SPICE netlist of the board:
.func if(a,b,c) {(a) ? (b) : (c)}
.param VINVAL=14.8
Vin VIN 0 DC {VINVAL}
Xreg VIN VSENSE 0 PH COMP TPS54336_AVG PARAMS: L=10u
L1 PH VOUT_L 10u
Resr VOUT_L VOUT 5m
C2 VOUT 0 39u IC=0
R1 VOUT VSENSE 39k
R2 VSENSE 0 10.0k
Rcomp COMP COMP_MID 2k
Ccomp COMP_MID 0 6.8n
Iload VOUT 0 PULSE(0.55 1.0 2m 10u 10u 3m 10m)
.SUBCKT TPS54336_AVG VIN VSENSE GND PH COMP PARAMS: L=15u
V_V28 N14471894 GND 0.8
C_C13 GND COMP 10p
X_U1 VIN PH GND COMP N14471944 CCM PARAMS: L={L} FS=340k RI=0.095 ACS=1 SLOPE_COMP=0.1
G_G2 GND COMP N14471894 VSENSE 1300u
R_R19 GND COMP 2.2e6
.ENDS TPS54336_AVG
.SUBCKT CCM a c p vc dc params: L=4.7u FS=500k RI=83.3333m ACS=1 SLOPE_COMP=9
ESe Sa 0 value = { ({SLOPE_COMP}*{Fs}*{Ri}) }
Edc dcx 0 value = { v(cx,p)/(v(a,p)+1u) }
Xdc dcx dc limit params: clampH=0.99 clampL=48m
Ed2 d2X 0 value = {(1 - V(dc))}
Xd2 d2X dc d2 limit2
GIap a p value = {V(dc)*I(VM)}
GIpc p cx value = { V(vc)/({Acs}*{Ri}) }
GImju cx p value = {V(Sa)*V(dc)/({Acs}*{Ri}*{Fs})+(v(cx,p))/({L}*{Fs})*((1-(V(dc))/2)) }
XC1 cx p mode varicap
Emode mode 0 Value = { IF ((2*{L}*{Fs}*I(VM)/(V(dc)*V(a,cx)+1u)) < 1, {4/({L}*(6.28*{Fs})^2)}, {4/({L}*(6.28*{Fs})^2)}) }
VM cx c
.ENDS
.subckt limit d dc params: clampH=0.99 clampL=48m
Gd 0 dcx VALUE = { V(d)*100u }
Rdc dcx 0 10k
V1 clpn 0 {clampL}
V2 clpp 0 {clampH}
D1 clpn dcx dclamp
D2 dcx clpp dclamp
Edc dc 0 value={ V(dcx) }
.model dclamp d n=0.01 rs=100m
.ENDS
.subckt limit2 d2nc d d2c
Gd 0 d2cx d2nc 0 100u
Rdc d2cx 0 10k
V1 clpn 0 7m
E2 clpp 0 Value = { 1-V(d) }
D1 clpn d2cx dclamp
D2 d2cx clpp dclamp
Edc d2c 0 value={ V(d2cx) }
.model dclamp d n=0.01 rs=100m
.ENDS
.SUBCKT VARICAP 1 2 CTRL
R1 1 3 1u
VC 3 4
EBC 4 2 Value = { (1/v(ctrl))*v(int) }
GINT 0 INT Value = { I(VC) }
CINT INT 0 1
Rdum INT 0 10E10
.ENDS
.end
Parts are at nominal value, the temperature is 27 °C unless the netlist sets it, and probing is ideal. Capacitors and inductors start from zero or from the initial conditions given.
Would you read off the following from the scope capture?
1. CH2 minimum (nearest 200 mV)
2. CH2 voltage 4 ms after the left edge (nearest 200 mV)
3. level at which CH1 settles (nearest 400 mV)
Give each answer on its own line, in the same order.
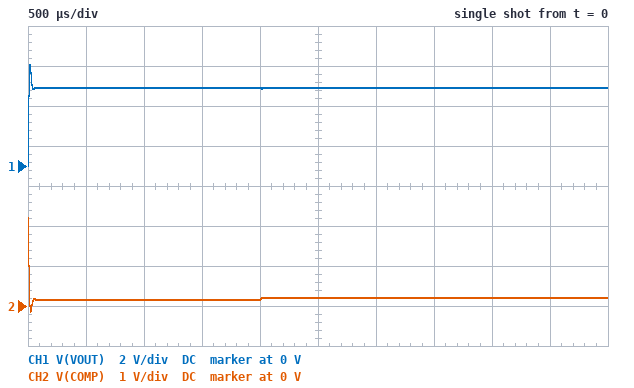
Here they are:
-200 mV
200 mV
4.0 V
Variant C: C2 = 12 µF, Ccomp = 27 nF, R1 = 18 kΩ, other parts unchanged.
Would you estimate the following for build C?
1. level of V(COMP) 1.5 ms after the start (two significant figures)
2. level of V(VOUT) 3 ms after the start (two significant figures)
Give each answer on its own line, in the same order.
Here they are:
110 mV
2.2 V
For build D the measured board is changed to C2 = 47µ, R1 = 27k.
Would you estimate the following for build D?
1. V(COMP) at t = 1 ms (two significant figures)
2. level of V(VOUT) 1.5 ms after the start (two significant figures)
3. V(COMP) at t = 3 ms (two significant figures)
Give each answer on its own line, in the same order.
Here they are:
130 mV
3.0 V
170 mV
